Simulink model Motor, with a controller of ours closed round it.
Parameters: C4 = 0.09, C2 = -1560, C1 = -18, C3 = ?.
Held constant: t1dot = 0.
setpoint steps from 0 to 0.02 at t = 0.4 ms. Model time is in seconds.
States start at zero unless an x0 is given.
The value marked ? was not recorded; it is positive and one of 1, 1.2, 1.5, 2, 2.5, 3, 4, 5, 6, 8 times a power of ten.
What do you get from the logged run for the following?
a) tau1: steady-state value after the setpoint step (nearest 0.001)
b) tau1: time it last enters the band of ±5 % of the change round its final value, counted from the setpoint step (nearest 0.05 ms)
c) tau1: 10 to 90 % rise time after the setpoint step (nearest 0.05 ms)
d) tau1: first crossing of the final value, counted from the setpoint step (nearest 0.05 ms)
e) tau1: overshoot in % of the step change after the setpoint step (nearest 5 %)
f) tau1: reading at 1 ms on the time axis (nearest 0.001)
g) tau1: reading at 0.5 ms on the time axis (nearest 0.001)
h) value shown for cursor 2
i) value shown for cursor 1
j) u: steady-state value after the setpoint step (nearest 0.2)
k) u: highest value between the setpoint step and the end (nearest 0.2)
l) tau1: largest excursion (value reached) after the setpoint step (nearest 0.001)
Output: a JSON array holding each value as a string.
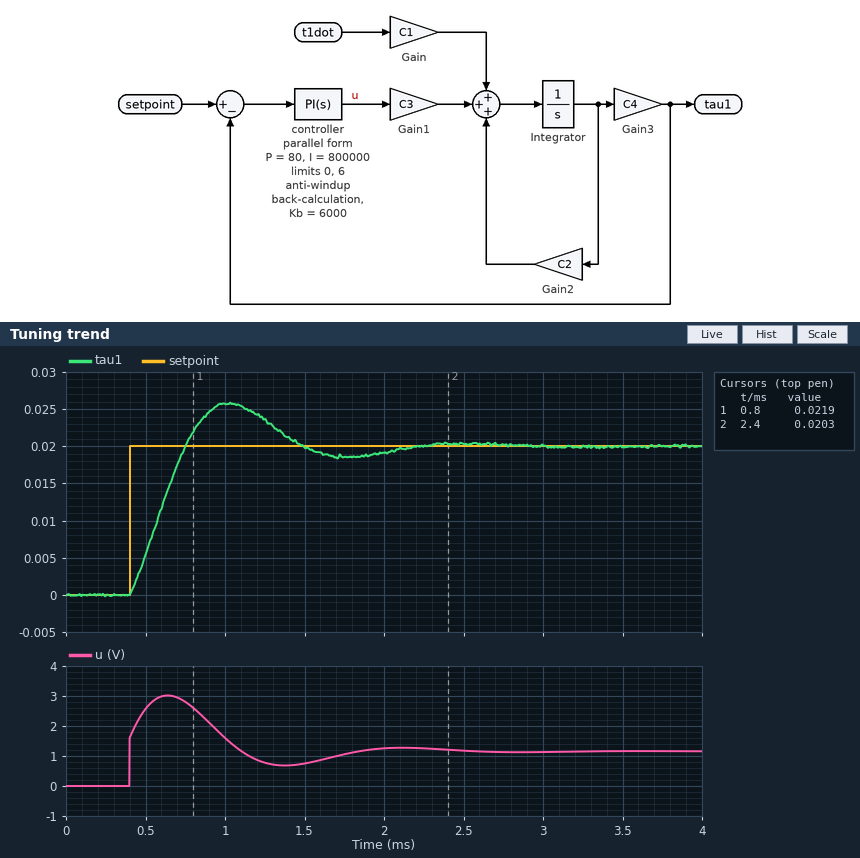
["0.020", "1.55 ms", "0.25 ms", "0.35 ms", "30 %", "0.026", "0.005", "0.0203", "0.0219", "1.2", "3.0", "0.026"]
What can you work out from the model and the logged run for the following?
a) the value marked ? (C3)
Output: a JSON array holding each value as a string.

["300"]
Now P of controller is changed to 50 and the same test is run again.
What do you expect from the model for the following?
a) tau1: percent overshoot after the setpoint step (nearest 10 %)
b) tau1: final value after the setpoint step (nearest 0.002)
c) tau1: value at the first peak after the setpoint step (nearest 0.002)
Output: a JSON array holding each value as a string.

["40 %", "0.020", "0.028"]
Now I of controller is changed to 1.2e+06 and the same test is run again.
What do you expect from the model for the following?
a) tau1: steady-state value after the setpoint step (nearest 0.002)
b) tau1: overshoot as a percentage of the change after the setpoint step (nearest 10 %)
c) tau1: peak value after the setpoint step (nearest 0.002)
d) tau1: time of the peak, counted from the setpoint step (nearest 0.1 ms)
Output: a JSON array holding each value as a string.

["0.020", "40 %", "0.028", "0.5 ms"]
